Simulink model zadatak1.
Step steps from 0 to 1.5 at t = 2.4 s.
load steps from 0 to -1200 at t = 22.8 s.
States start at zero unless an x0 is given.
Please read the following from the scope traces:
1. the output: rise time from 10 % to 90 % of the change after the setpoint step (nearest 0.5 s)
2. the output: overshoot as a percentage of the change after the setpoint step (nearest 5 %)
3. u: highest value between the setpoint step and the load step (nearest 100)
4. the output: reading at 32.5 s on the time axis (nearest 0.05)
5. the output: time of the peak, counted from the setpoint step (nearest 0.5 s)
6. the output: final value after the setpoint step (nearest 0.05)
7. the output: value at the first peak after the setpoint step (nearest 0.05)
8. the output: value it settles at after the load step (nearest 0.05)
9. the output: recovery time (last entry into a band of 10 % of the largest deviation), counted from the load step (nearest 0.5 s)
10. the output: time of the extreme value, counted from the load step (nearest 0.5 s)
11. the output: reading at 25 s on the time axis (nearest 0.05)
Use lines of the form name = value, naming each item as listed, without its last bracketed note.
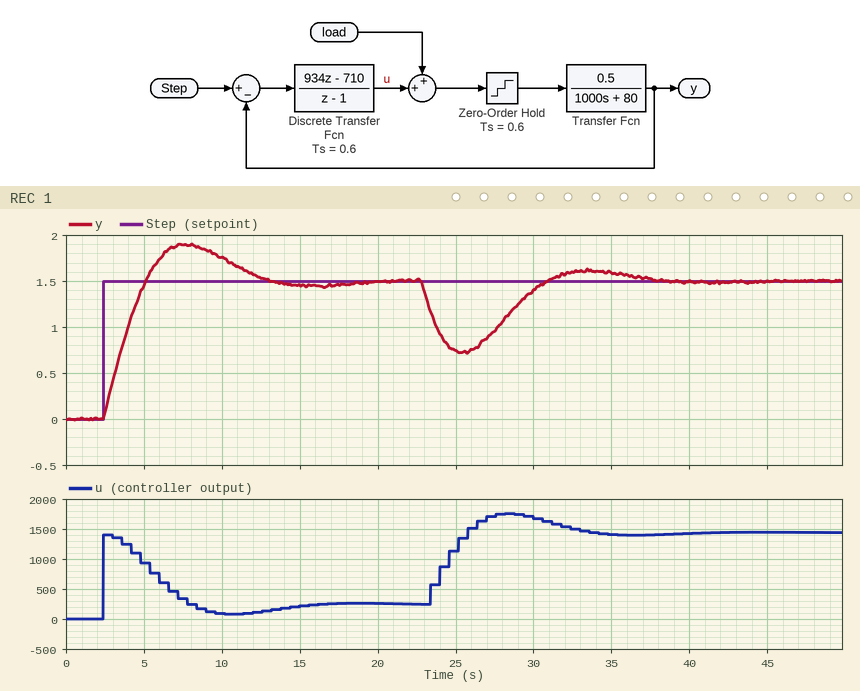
the output: rise time from 10 % to 90 % of the change after the setpoint step = 2.0 s
the output: overshoot as a percentage of the change after the setpoint step = 25 %
u: highest value between the setpoint step and the load step = 1400
the output: reading at 32.5 s on the time axis = 1.60
the output: time of the peak, counted from the setpoint step = 5.5 s
the output: final value after the setpoint step = 1.50
the output: value at the first peak after the setpoint step = 1.90
the output: value it settles at after the load step = 1.50
the output: recovery time (last entry into a band of 10 % of the largest deviation), counted from the load step = 12.5 s
the output: time of the extreme value, counted from the load step = 2.5 s
the output: reading at 25 s on the time axis = 0.75
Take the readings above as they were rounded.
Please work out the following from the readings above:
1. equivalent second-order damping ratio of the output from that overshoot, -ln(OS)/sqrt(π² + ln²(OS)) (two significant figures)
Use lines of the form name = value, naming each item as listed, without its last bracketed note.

equivalent second-order damping ratio of the output from that overshoot, -ln(OS)/sqrt(π² + ln²(OS)) = 0.40
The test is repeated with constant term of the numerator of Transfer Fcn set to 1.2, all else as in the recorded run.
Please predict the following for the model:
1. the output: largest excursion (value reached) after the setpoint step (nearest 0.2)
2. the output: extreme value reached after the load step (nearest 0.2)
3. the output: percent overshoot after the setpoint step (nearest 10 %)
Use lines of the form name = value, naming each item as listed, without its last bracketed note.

the output: largest excursion (value reached) after the setpoint step = 1.8
the output: extreme value reached after the load step = 0.4
the output: percent overshoot after the setpoint step = 20 %
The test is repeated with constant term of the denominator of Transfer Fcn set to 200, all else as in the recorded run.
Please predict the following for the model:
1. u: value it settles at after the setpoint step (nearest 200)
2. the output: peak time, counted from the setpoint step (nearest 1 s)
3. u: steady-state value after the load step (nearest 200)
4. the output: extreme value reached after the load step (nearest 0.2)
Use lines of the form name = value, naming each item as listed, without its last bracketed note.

u: value it settles at after the setpoint step = 600
the output: peak time, counted from the setpoint step = 6 s
u: steady-state value after the load step = 1800
the output: extreme value reached after the load step = 0.8
